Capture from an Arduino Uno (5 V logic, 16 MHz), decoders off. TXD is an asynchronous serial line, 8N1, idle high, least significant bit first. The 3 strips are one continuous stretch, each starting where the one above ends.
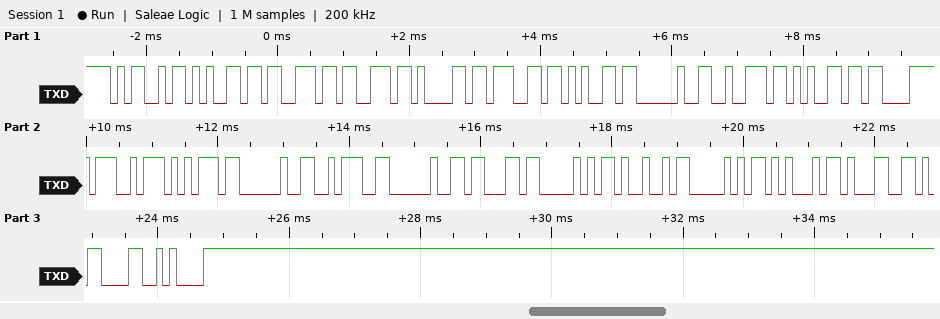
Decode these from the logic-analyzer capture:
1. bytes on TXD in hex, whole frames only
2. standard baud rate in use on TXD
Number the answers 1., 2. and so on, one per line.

1. 4D 65 73 73 61 67 65 20 72 65 C3 A7 75 20 3A 20 63 50 49 50 45 31 0D 0A
2. 9600 baud
